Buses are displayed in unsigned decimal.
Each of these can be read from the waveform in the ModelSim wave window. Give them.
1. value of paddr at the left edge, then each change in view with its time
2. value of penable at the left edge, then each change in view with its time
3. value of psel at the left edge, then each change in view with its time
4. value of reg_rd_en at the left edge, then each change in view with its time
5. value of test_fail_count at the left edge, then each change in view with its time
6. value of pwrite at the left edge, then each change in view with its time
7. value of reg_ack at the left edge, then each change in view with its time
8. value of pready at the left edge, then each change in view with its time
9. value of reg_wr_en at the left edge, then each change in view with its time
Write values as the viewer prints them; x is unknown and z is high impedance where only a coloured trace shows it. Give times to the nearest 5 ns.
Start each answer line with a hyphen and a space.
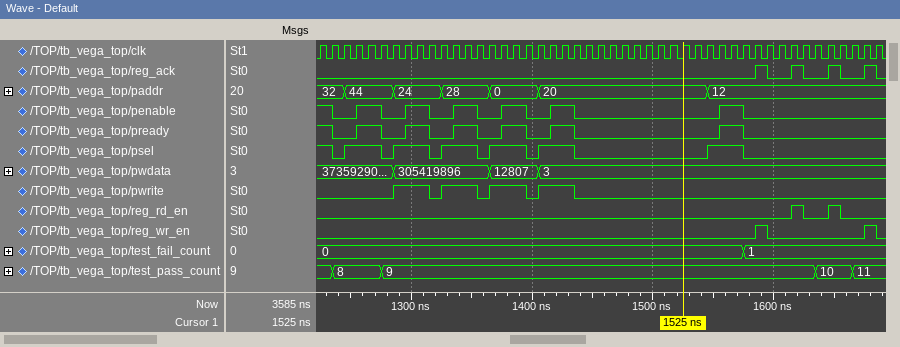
- 32, 44 at 1245 ns, 24 at 1285 ns, 28 at 1325 ns, 0 at 1365 ns, 20 at 1405 ns, 12 at 1545 ns
- 1, 0 at 1235 ns, 1 at 1255 ns, 0 at 1275 ns, 1 at 1295 ns, 0 at 1315 ns, 1 at 1335 ns, 0 at 1355 ns, 1 at 1375 ns, 0 at 1395 ns, 1 at 1415 ns, 0 at 1435 ns, 1 at 1555 ns, 0 at 1575 ns
- 1, 0 at 1235 ns, 1 at 1245 ns, 0 at 1275 ns, 1 at 1285 ns, 0 at 1315 ns, 1 at 1325 ns, 0 at 1355 ns, 1 at 1365 ns, 0 at 1395 ns, 1 at 1405 ns, 0 at 1435 ns, 1 at 1545 ns, 0 at 1575 ns
- 0, 1 at 1615 ns, 0 at 1625 ns, 1 at 1645 ns, 0 at 1655 ns
- 0, 1 at 1575 ns
- 0, 1 at 1285 ns, 0 at 1315 ns, 1 at 1325 ns, 0 at 1355 ns, 1 at 1365 ns, 0 at 1395 ns, 1 at 1405 ns, 0 at 1435 ns
- 0, 1 at 1585 ns, 0 at 1595 ns, 1 at 1615 ns, 0 at 1625 ns, 1 at 1645 ns, 0 at 1655 ns, 1 at 1675 ns, 0 at 1685 ns
- 1, 0 at 1235 ns, 1 at 1255 ns, 0 at 1275 ns, 1 at 1295 ns, 0 at 1315 ns, 1 at 1335 ns, 0 at 1355 ns, 1 at 1375 ns, 0 at 1395 ns, 1 at 1415 ns, 0 at 1435 ns, 1 at 1555 ns, 0 at 1575 ns
- 0, 1 at 1585 ns, 0 at 1595 ns, 1 at 1675 ns, 0 at 1685 ns
